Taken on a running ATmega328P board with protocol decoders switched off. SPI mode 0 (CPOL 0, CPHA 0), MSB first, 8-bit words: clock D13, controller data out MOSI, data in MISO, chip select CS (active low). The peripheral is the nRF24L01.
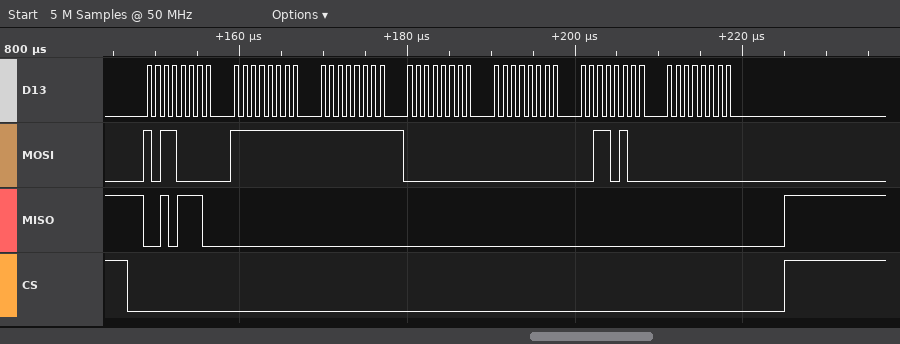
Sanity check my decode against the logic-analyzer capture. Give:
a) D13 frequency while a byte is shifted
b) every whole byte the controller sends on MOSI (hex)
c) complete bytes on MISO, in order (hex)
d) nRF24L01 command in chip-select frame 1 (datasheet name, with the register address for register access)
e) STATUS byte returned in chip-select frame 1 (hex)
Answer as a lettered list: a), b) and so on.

a) 1 MHz
b) B0 FF FF 00 00 34 00
c) 2E 00 00 00 00 00 00
d) W_TX_PAYLOAD_NOACK
e) 0x2E
